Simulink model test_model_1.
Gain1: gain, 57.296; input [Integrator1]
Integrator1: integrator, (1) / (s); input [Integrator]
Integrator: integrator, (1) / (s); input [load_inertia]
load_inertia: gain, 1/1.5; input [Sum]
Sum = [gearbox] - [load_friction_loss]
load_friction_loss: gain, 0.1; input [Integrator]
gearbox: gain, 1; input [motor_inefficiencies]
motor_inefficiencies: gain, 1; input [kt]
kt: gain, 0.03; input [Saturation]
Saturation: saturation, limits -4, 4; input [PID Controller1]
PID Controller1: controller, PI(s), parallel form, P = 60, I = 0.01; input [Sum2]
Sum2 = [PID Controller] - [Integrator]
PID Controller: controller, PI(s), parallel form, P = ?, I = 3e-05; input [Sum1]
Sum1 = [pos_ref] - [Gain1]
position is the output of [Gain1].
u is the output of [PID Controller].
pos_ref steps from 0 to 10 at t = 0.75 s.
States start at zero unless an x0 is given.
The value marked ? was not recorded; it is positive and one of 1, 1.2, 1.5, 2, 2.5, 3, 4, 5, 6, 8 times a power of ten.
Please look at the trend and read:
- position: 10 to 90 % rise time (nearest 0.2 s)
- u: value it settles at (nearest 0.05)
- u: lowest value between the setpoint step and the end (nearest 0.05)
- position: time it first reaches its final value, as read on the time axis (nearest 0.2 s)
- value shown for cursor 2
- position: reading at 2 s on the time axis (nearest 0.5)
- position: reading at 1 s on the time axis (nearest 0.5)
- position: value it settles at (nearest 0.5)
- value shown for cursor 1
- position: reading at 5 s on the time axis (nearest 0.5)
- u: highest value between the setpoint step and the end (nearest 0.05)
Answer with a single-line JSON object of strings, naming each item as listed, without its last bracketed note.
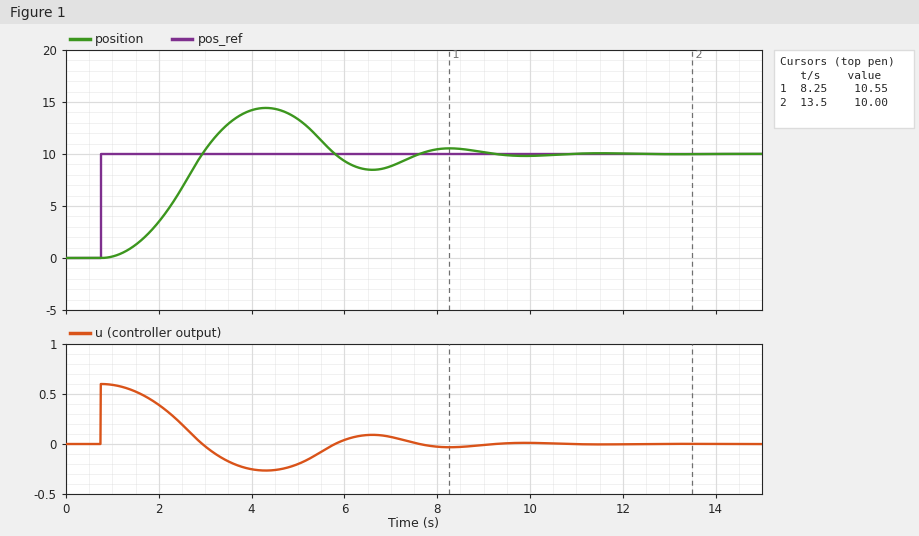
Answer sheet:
{"position: 10 to 90 % rise time": "1.4 s", "u: value it settles at": "0.00", "u: lowest value between the setpoint step and the end": "-0.25", "position: time it first reaches its final value, as read on the time axis": "3.0 s", "value shown for cursor 2": "10.00", "position: reading at 2 s on the time axis": "3.5", "position: reading at 1 s on the time axis": "0.0", "position: value it settles at": "10.0", "value shown for cursor 1": "10.55", "position: reading at 5 s on the time axis": "13.5", "u: highest value between the setpoint step and the end": "0.60"}
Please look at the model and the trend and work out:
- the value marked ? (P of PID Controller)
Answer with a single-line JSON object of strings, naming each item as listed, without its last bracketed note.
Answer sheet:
{"the value marked ?": "0.06"}
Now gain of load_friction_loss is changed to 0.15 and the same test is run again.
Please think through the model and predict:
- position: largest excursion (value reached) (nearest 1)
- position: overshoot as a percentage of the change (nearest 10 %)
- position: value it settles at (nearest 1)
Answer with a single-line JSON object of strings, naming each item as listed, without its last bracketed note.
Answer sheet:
{"position: largest excursion (value reached)": "14", "position: overshoot as a percentage of the change": "40 %", "position: value it settles at": "10"}
